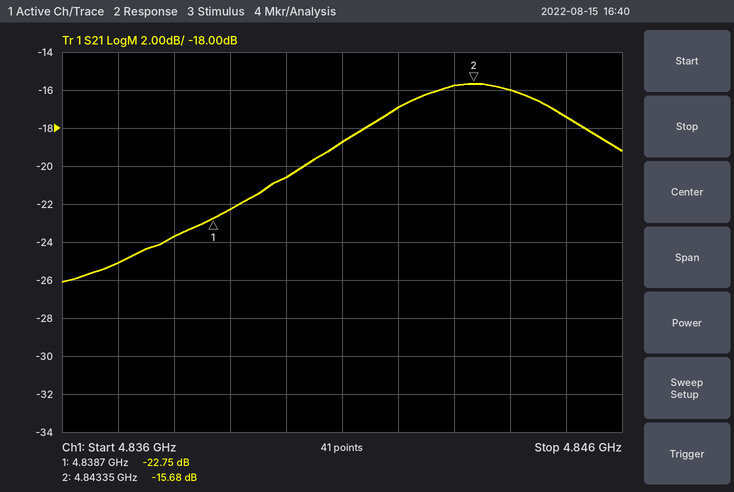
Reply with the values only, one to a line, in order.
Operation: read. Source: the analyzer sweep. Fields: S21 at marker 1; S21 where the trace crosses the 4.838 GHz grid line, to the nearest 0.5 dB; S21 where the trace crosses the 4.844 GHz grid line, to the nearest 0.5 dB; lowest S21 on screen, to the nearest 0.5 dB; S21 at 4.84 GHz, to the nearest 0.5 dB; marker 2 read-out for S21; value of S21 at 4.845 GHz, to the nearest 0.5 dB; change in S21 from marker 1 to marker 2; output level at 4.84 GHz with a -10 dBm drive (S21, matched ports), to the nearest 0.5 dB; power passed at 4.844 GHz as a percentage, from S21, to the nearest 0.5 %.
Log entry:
-22.75 dB
-23.5 dB
-16.0 dB
-26.0 dB
-20.5 dB
-15.68 dB
-17.5 dB
7.07 dB
-30.5 dBm
2.5 %
